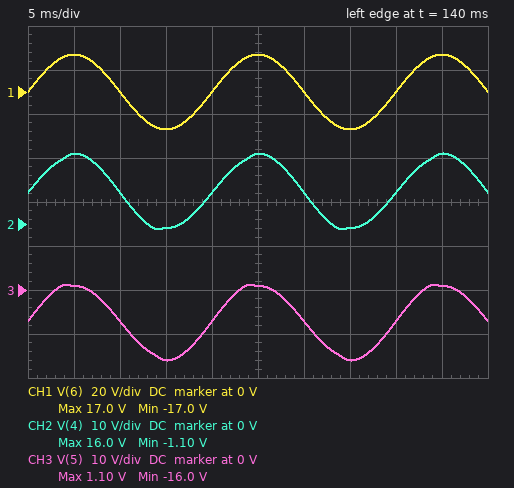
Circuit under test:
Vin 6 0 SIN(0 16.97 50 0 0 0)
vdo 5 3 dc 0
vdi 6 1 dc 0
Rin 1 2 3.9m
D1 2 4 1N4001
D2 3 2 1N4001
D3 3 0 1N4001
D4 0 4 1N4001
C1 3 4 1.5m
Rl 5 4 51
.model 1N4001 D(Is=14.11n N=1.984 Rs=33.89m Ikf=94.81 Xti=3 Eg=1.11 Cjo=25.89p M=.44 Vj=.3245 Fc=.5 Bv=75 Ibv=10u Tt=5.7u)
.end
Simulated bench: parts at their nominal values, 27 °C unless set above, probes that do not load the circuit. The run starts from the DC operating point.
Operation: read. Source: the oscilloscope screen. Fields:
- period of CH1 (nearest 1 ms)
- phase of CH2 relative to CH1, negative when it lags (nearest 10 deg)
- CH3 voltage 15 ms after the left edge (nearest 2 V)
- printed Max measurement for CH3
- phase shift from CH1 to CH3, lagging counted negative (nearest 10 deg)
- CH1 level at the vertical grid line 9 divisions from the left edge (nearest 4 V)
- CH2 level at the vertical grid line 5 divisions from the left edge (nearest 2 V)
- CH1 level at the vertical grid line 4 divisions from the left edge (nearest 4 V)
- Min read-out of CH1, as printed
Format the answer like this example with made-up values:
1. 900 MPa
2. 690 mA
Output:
1. 20 ms
2. 0 deg
3. -16 V
4. 1.10 V
5. 0 deg
6. 16 V
7. 16 V
8. 0 V
9. -17.0 V
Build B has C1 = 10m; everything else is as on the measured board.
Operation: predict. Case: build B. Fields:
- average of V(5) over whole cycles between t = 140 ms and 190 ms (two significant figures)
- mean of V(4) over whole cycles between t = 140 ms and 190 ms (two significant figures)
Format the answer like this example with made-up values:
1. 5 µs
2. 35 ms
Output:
1. -7.4 V
2. 7.4 V
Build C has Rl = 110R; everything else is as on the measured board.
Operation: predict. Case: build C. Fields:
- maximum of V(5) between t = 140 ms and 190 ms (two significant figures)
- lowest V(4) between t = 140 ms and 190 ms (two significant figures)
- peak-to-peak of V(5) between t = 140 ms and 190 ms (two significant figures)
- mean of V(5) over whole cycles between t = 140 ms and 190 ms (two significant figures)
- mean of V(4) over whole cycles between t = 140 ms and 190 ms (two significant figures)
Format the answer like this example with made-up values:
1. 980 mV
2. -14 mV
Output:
1. 1.0 V
2. -1.0 V
3. 17 V
4. -7.4 V
5. 7.4 V
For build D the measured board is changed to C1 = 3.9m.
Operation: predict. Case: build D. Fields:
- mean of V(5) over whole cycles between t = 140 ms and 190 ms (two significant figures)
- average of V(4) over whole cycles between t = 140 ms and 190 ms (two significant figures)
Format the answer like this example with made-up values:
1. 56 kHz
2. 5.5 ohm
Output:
1. -7.3 V
2. 7.3 V
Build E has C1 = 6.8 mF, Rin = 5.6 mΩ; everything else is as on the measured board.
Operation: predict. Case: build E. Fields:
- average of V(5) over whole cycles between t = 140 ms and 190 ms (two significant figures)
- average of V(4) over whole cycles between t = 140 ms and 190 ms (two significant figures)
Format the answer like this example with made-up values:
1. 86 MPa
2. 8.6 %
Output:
1. -7.4 V
2. 7.4 V
